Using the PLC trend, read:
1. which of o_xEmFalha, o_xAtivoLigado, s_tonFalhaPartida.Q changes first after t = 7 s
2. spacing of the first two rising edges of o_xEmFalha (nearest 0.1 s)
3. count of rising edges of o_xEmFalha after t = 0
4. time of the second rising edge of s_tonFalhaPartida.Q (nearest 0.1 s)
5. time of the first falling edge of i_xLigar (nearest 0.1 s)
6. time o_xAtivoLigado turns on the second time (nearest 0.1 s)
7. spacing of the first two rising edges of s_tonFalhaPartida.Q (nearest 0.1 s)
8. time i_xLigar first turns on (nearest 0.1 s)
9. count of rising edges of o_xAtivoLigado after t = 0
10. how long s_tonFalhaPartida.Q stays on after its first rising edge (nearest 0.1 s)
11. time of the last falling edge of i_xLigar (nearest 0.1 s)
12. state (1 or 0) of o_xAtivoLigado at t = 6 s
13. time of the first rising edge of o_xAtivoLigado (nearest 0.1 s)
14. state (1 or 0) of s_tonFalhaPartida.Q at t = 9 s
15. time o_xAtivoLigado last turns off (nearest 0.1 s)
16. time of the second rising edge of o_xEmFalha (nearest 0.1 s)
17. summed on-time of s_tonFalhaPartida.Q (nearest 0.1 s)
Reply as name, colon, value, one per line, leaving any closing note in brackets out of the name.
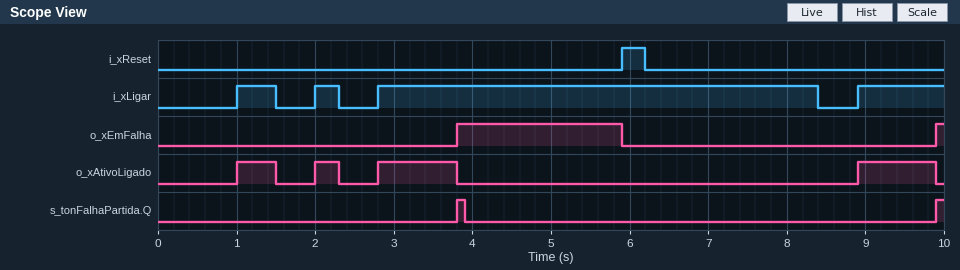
which of o_xEmFalha, o_xAtivoLigado, s_tonFalhaPartida.Q changes first after t = 7 s: o_xAtivoLigado
spacing of the first two rising edges of o_xEmFalha: 6.1 s
count of rising edges of o_xEmFalha after t = 0: 2
time of the second rising edge of s_tonFalhaPartida.Q: 9.9 s
time of the first falling edge of i_xLigar: 1.5 s
time o_xAtivoLigado turns on the second time: 2.0 s
spacing of the first two rising edges of s_tonFalhaPartida.Q: 6.1 s
time i_xLigar first turns on: 1.0 s
count of rising edges of o_xAtivoLigado after t = 0: 4
how long s_tonFalhaPartida.Q stays on after its first rising edge: 0.1 s
time of the last falling edge of i_xLigar: 8.4 s
state (1 or 0) of o_xAtivoLigado at t = 6 s: 0
time of the first rising edge of o_xAtivoLigado: 1.0 s
state (1 or 0) of s_tonFalhaPartida.Q at t = 9 s: 0
time o_xAtivoLigado last turns off: 9.9 s
time of the second rising edge of o_xEmFalha: 9.9 s
summed on-time of s_tonFalhaPartida.Q: 0.2 s
